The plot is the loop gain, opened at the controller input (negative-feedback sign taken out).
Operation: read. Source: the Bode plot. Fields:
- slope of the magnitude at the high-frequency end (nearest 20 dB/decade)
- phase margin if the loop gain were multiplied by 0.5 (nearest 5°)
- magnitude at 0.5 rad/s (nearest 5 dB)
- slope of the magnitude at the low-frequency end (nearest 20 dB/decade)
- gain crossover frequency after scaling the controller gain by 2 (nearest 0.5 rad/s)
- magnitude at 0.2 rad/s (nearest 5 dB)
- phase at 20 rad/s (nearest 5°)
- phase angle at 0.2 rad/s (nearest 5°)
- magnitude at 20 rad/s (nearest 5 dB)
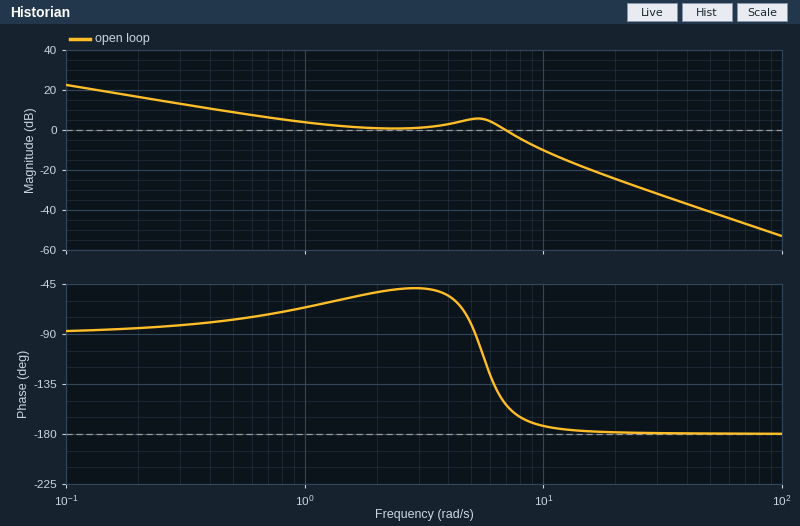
-40 dB/decade
110°
10 dB
-20 dB/decade
8.5 rad/s
15 dB
-180°
-85°
-25 dB
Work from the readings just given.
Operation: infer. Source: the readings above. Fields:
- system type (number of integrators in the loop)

1
